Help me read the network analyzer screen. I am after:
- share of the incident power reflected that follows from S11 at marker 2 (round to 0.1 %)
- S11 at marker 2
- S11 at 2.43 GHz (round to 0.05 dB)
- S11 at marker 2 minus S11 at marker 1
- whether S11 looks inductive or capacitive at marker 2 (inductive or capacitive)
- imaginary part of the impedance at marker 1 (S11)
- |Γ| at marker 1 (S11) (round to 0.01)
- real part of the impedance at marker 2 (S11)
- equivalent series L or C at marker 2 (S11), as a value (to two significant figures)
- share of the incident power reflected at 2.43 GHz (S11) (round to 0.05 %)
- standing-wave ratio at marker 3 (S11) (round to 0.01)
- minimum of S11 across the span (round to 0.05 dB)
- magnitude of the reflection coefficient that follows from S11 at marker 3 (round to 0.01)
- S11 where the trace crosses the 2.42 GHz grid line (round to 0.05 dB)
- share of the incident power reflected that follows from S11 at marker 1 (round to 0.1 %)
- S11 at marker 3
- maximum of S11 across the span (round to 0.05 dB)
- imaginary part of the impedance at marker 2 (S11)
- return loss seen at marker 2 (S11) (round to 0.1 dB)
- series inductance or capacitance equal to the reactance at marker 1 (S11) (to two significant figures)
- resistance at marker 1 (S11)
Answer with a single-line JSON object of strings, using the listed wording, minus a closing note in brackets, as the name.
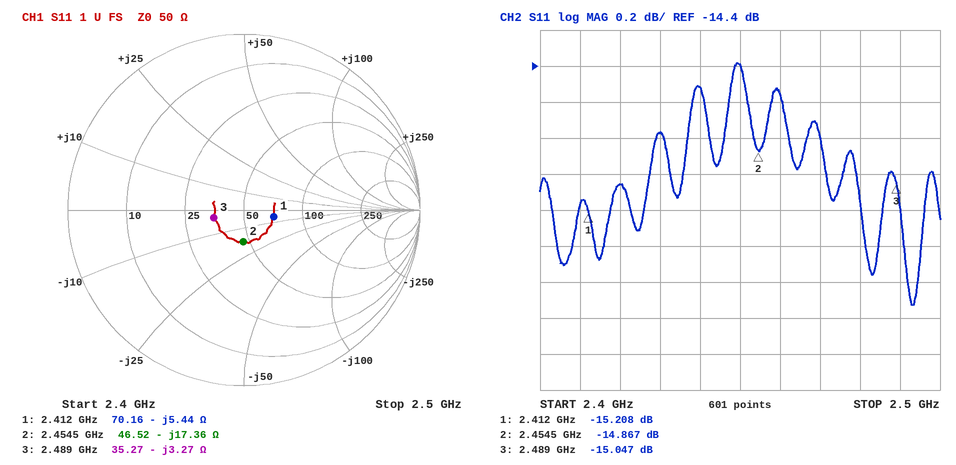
{"share of the incident power reflected that follows from S11 at marker 2": "3.3 %", "S11 at marker 2": "-14.867 dB", "S11 at 2.43 GHz": "-14.75 dB", "S11 at marker 2 minus S11 at marker 1": "0.341 dB", "whether S11 looks inductive or capacitive at marker 2": "capacitive", "imaginary part of the impedance at marker 1": "-5.44 Ω", "|Γ| at marker 1 (S11)": "0.17", "real part of the impedance at marker 2": "46.52 Ω", "equivalent series L or C at marker 2 (S11), as a value": "3.7 pF", "share of the incident power reflected at 2.43 GHz (S11)": "3.35 %", "standing-wave ratio at marker 3 (S11)": "1.43", "minimum of S11 across the span": "-15.75 dB", "magnitude of the reflection coefficient that follows from S11 at marker 3": "0.18", "S11 where the trace crosses the 2.42 GHz grid line": "-15.05 dB", "share of the incident power reflected that follows from S11 at marker 1": "3.0 %", "S11 at marker 3": "-15.047 dB", "maximum of S11 across the span": "-14.40 dB", "imaginary part of the impedance at marker 2": "-17.36 Ω", "return loss seen at marker 2 (S11)": "14.9 dB", "series inductance or capacitance equal to the reactance at marker 1 (S11)": "12 pF", "resistance at marker 1": "70.16 Ω"}
